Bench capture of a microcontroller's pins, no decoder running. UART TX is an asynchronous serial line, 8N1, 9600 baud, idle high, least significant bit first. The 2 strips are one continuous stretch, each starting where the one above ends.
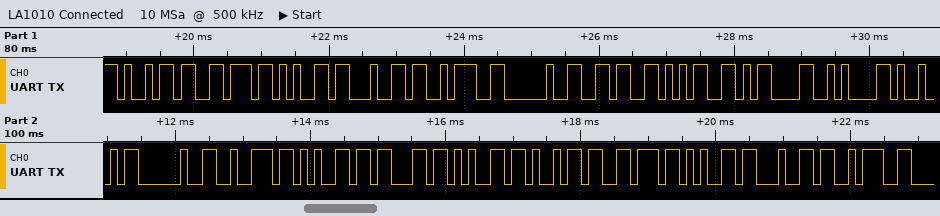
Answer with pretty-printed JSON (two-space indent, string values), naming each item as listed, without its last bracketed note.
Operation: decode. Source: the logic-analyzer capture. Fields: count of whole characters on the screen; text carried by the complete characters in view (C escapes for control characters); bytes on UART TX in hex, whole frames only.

{
  "count of whole characters on the screen": "21",
  "text carried by the complete characters in view": "\"ived: 65\\r\\nI received:\"",
  "bytes on UART TX in hex, whole frames only": "69 76 65 64 3A 20 36 35 0D 0A 49 20 72 65 63 65 69 76 65 64 3A"
}
